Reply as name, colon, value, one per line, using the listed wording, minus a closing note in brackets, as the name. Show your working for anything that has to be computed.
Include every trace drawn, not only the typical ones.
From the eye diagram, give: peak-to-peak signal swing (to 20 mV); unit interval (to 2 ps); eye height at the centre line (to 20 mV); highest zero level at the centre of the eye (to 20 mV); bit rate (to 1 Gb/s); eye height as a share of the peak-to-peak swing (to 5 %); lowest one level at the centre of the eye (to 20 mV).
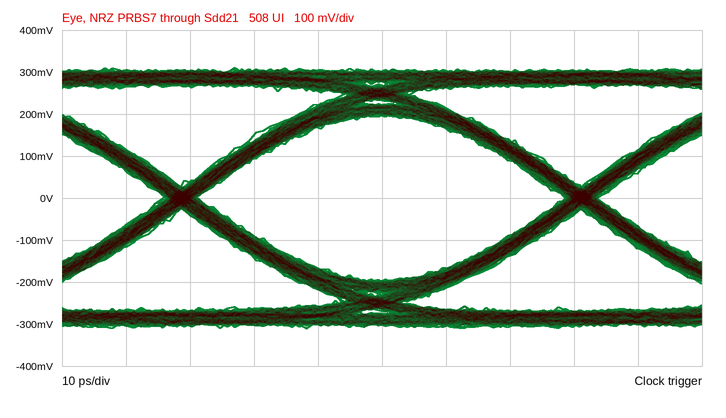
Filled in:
peak-to-peak signal swing: 620 mV
unit interval: 62 ps
eye height at the centre line: 400 mV
highest zero level at the centre of the eye: -200 mV
bit rate: 16 Gb/s
eye height as a share of the peak-to-peak swing: 400 mV / 620 mV ≈ 65 %
lowest one level at the centre of the eye: 200 mV
